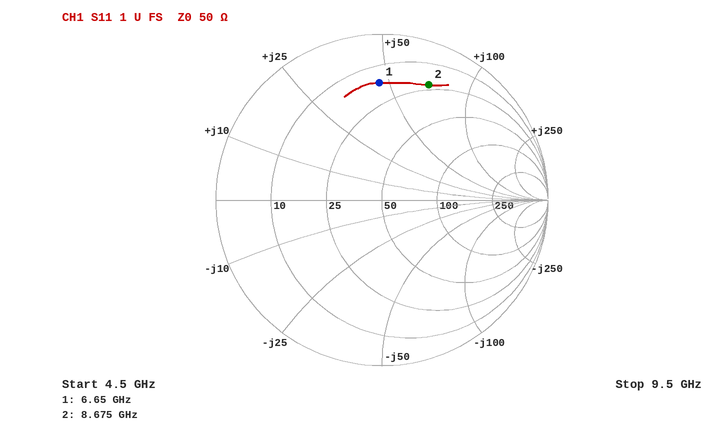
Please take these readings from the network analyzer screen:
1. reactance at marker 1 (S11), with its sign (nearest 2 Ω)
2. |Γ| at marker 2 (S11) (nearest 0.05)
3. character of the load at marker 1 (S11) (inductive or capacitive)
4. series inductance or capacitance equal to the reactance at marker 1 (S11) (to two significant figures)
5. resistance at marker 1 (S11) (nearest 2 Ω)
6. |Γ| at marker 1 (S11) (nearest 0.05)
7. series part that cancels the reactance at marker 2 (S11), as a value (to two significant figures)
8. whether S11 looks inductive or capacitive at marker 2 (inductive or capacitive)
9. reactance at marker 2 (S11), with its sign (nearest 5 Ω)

+46 Ω
0.75
inductive
1.1 nH
16 Ω
0.70
260 fF
inductive
+70 Ω
